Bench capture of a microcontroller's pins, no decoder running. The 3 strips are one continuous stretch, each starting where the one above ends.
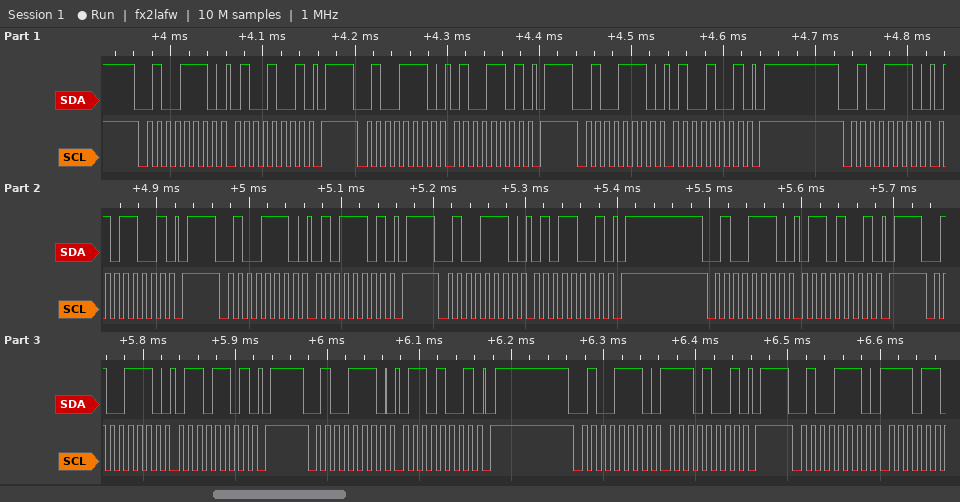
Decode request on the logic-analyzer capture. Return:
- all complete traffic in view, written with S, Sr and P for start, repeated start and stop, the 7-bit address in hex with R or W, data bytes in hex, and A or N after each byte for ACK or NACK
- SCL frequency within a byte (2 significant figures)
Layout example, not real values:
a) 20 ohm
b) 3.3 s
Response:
a) S 27W A 49 A P S 27W A 4D A P S 27W A 49 A P S 27W A 59 A P S 27W A 5D A P S 27W A 59 A P S 27W A 69 A P S 27W A 6D A P S 27W A 69 A P S 27W A E9 A P S 27W A
b) 100 kHz
